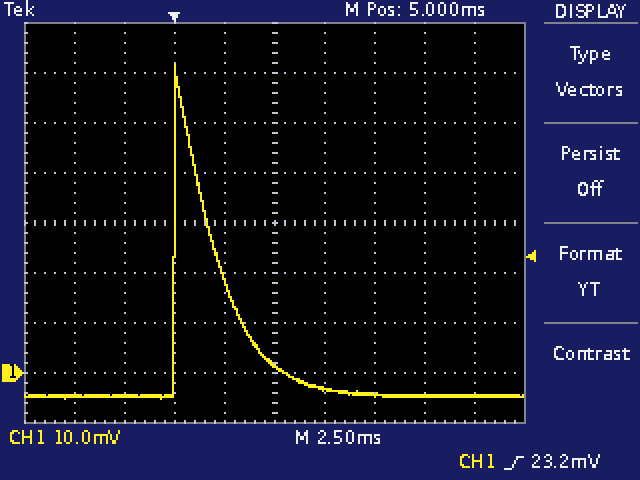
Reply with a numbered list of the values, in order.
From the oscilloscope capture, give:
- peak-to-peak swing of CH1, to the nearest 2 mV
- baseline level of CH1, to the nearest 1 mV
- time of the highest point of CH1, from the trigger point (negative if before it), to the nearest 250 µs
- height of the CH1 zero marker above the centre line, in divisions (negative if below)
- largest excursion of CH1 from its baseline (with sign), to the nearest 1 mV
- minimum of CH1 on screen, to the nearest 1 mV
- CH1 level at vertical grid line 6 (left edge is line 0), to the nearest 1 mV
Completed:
1. 66 mV
2. -5 mV
3. 0.00 ms
4. -3.0 div
5. +66 mV
6. -5 mV
7. -3 mV
